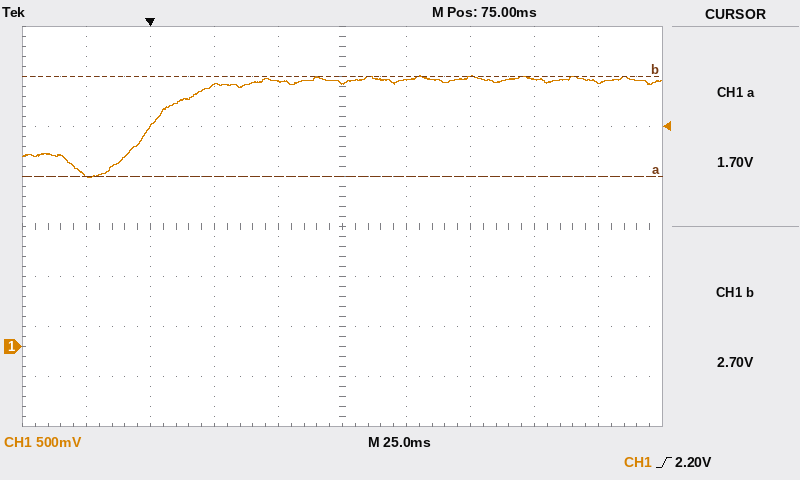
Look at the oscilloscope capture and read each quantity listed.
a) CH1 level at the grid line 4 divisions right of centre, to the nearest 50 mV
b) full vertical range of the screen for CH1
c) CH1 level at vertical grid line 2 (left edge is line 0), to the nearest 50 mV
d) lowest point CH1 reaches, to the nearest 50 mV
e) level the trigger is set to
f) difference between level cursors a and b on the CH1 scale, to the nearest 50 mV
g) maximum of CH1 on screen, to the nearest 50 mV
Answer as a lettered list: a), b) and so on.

a) 2.65 V
b) 4 V
c) 2.20 V
d) 1.70 V
e) 2.20 V
f) 1.00 V
g) 2.70 V
